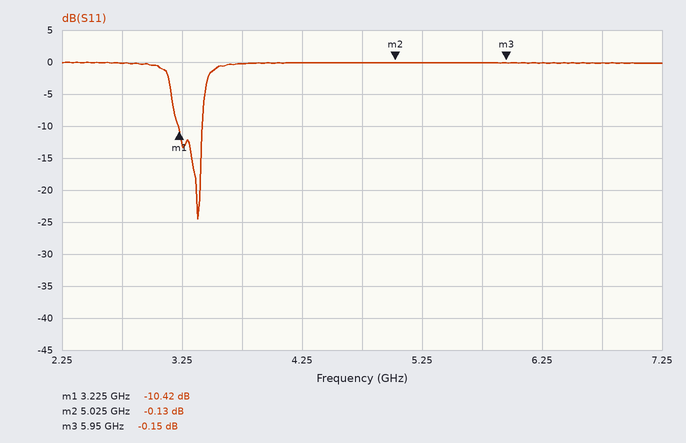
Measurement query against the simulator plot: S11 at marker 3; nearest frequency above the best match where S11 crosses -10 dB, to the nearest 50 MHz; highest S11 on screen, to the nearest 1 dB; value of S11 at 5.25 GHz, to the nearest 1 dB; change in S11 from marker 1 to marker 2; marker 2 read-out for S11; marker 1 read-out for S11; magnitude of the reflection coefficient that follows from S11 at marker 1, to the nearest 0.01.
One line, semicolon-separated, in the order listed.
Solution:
-0.15 dB; 3.40 GHz; 0 dB; 0 dB; 10.29 dB; -0.13 dB; -10.42 dB; 0.30
